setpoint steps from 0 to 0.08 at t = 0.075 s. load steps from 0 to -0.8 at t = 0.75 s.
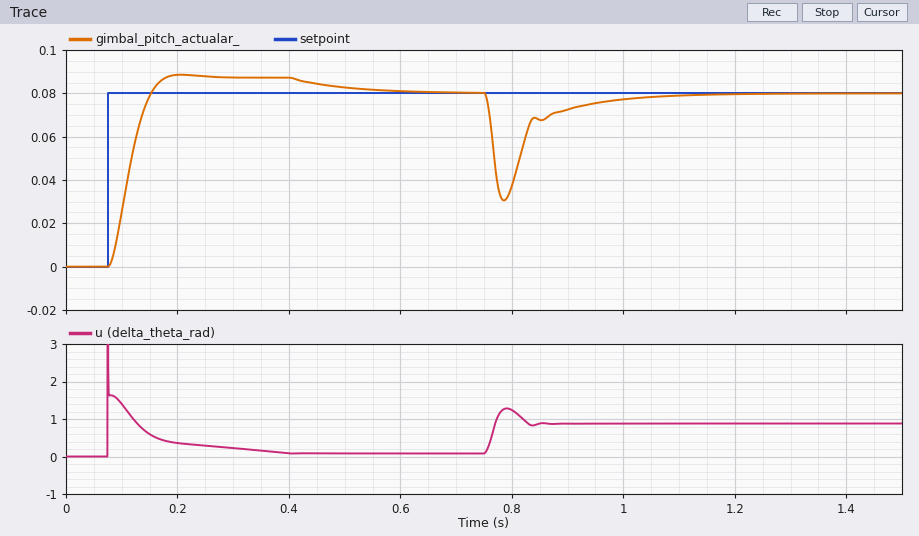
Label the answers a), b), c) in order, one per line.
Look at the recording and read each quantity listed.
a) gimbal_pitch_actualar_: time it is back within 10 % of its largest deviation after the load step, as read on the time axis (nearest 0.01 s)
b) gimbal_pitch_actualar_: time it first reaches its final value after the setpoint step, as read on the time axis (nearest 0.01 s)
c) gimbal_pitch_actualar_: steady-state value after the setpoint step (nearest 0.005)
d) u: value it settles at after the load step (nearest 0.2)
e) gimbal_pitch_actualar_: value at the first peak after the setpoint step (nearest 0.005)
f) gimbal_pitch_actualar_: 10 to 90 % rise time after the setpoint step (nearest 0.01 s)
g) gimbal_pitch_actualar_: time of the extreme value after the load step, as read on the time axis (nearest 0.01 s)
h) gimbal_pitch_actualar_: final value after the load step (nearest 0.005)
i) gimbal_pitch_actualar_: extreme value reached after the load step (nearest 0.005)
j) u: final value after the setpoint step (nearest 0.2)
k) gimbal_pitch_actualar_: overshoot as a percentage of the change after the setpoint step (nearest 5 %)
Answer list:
a) 0.94 s
b) 0.15 s
c) 0.080
d) 0.8
e) 0.090
f) 0.05 s
g) 0.79 s
h) 0.080
i) 0.030
j) 0.0
k) 10 %
